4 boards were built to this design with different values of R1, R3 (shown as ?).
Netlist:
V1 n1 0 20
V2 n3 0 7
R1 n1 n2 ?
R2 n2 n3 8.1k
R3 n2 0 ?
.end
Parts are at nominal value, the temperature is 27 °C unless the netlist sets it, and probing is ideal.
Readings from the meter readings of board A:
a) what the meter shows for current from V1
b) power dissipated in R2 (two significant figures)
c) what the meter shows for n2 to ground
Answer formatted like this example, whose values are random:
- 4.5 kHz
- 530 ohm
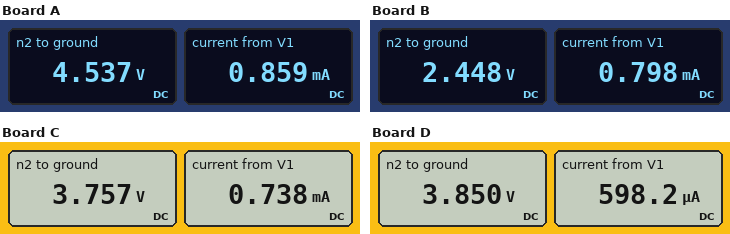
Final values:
- 0.859 mA
- 750 µW
- 4.537 V
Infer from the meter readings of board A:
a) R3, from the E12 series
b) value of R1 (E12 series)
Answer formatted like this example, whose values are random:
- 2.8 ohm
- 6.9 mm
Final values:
- 3.9 kΩ
- 18 kΩ
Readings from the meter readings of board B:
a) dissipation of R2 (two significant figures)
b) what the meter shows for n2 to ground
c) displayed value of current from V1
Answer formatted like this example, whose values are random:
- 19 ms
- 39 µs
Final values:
- 2.6 mW
- 2.448 V
- 0.798 mA
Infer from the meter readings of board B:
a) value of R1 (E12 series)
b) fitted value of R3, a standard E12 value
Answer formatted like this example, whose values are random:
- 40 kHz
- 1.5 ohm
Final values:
- 22 kΩ
- 1.8 kΩ
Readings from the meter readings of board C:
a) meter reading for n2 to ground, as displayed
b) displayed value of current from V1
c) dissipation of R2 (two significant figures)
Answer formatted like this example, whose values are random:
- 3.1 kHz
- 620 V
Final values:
- 3.757 V
- 0.738 mA
- 1.3 mW
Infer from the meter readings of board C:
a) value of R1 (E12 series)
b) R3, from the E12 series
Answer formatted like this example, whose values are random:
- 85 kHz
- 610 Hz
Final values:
- 22 kΩ
- 3.3 kΩ
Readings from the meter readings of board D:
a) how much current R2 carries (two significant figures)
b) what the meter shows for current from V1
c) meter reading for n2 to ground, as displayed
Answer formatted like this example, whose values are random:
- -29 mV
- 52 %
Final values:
- 390 µA
- 598.2 µA
- 3.850 V
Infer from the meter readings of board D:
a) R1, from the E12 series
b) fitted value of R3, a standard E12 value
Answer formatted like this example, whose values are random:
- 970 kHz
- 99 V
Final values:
- 27 kΩ
- 3.9 kΩ
